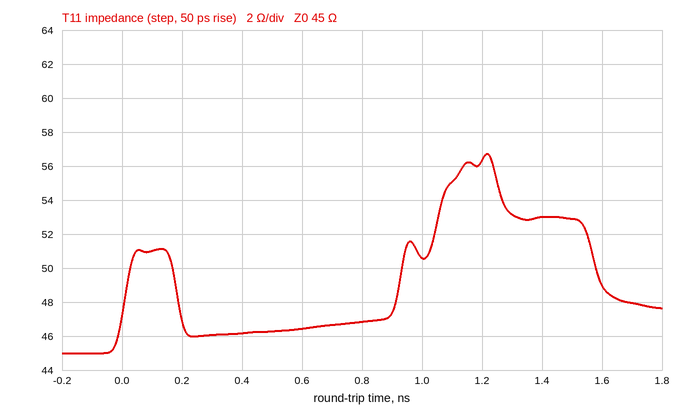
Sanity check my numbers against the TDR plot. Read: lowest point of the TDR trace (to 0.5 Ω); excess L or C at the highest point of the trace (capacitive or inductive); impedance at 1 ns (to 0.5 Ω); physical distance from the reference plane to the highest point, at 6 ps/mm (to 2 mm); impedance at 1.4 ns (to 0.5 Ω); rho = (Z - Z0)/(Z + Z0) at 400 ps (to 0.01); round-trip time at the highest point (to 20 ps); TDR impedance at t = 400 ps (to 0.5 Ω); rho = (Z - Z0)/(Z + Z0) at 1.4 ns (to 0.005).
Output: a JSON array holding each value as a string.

["45.0 Ω", "inductive", "50.5 Ω", "102 mm", "53.0 Ω", "+0.01", "1.22 ns", "46.0 Ω", "+0.080"]
